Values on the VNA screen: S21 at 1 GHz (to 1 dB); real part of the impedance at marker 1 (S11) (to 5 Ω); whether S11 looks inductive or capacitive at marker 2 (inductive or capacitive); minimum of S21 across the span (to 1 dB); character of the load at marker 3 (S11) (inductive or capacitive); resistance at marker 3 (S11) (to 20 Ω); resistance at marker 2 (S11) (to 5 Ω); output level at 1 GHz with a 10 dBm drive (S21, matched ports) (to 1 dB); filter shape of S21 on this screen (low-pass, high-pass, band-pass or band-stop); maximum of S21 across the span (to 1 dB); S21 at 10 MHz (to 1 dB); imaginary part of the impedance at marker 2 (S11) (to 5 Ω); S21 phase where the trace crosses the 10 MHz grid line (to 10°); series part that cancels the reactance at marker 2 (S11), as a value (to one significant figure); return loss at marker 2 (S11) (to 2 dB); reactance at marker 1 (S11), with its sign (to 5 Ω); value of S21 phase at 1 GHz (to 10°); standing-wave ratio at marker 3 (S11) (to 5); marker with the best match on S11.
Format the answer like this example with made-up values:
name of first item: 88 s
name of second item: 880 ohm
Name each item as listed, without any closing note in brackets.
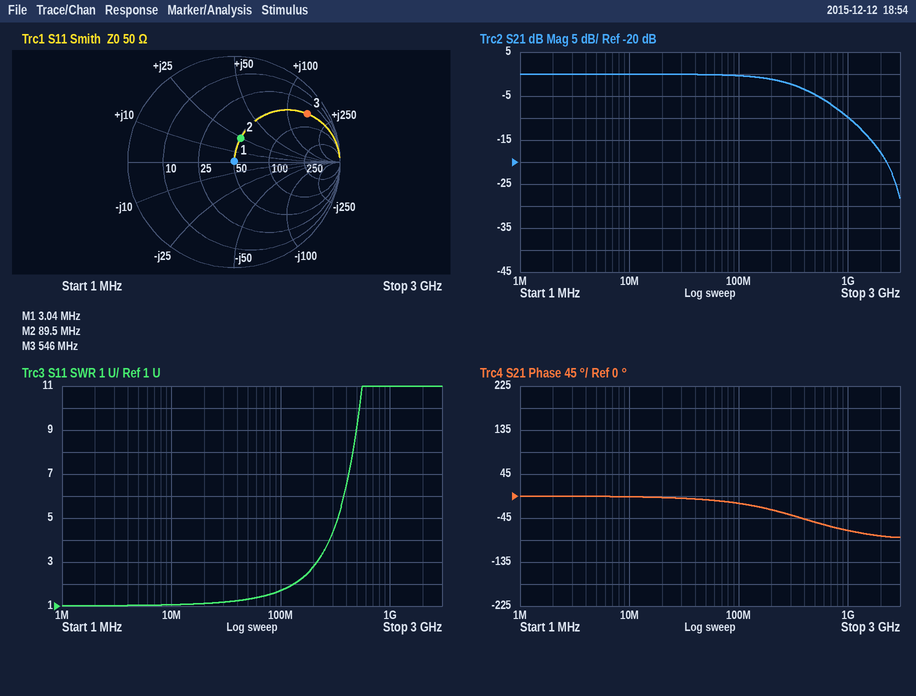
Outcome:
S21 at 1 GHz: -10 dB
real part of the impedance at marker 1 (S11): 50 Ω
whether S11 looks inductive or capacitive at marker 2: inductive
minimum of S21 across the span: -28 dB
character of the load at marker 3 (S11): inductive
resistance at marker 3 (S11): 60 Ω
resistance at marker 2 (S11): 50 Ω
output level at 1 GHz with a 10 dBm drive (S21, matched ports): 0 dBm
filter shape of S21 on this screen: low-pass
maximum of S21 across the span: 0 dB
S21 at 10 MHz: 0 dB
imaginary part of the impedance at marker 2 (S11): +25 Ω
S21 phase where the trace crosses the 10 MHz grid line: 0°
series part that cancels the reactance at marker 2 (S11), as a value: 70 pF
return loss at marker 2 (S11): 12 dB
reactance at marker 1 (S11), with its sign: 0 Ω
value of S21 phase at 1 GHz: -70°
standing-wave ratio at marker 3 (S11): 10
marker with the best match on S11: marker 1
